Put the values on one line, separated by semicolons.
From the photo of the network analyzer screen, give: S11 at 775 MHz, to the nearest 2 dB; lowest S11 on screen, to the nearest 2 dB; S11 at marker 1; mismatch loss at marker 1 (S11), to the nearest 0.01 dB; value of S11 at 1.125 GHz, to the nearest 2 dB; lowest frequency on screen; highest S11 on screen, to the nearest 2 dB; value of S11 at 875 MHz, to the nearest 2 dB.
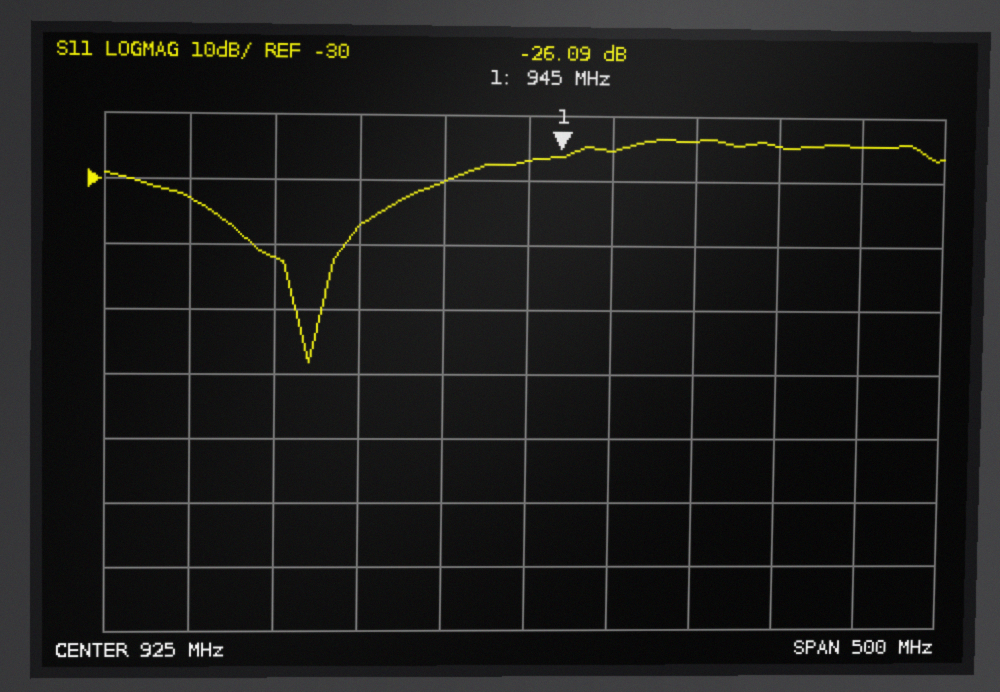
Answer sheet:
-42 dB; -58 dB; -26.09 dB; 0.01 dB; -24 dB; 675 MHz; -24 dB; -30 dB
